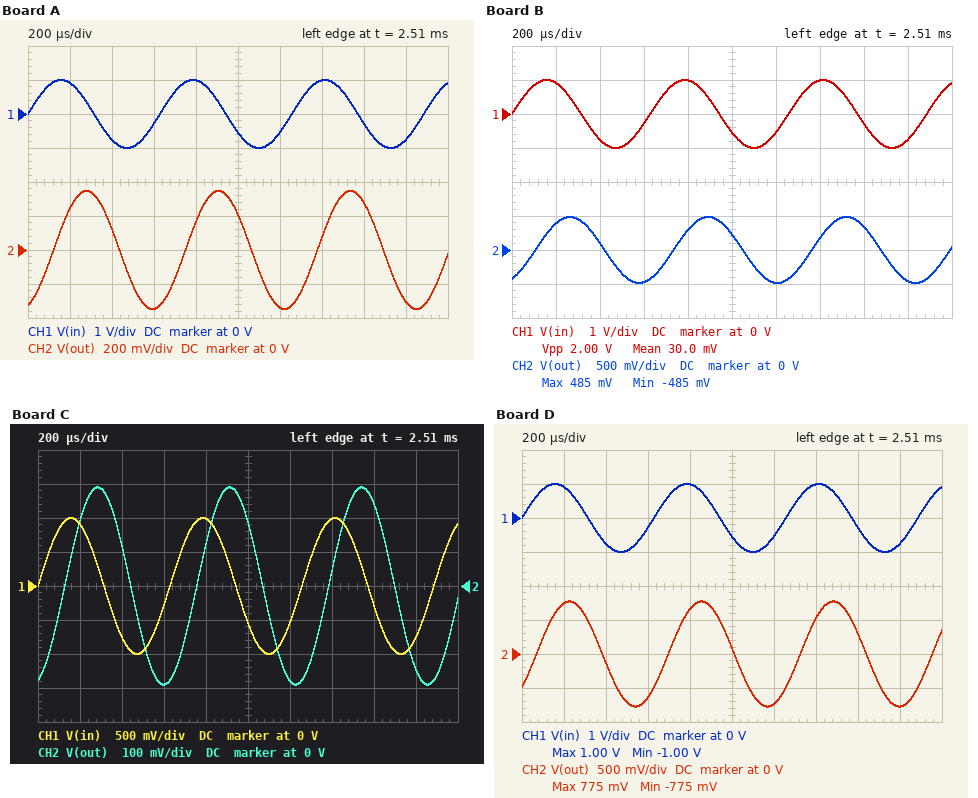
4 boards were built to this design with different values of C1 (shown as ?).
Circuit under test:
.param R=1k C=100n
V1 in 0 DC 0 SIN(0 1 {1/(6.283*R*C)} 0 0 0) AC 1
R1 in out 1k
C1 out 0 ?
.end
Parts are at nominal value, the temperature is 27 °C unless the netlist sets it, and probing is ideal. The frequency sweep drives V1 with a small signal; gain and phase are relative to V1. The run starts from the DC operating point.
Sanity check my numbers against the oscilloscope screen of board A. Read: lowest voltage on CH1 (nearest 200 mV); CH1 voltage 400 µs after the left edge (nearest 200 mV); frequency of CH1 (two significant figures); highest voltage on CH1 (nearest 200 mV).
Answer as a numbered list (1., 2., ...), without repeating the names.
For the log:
1. -1.0 V
2. -800 mV
3. 1.6 kHz
4. 1.0 V
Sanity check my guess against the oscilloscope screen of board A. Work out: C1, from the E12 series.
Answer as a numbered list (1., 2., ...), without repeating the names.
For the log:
1. 270 nF
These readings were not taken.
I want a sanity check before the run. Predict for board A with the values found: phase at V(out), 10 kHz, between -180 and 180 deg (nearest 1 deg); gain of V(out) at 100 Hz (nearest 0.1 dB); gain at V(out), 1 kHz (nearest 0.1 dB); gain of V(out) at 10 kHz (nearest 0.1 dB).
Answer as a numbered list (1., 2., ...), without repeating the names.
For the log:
1. -87 deg
2. -0.1 dB
3. -5.9 dB
4. -24.6 dB
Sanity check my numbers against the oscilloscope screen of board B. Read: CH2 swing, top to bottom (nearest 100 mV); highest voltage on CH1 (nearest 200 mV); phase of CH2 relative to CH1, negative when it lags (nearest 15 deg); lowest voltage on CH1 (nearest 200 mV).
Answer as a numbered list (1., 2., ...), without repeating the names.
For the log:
1. 1.0 V
2. 1.0 V
3. -60 deg
4. -1.0 V
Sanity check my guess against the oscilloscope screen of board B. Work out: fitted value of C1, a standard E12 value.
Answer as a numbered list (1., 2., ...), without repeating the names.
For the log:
1. 180 nF
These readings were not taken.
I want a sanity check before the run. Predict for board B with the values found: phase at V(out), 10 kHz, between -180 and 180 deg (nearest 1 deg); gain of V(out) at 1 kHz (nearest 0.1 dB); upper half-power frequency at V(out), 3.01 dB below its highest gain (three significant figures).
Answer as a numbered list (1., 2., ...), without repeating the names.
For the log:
1. -85 deg
2. -3.6 dB
3. 884 Hz
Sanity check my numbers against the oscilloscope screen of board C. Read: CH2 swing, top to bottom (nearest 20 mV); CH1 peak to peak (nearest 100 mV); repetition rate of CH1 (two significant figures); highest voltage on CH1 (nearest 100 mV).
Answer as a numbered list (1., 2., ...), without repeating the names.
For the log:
1. 580 mV
2. 2.0 V
3. 1.6 kHz
4. 1.0 V
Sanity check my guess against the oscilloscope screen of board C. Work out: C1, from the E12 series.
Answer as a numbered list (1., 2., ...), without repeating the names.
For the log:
1. 330 nF
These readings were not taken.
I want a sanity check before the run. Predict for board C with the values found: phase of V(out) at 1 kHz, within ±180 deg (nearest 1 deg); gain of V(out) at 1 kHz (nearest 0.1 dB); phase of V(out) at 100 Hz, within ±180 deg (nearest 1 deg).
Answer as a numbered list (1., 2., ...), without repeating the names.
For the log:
1. -64 deg
2. -7.2 dB
3. -12 deg
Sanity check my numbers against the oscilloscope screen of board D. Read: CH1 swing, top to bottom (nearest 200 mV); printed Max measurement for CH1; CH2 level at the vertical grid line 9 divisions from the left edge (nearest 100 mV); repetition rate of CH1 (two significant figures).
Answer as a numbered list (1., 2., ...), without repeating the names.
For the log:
1. 2.0 V
2. 1.00 V
3. -800 mV
4. 1.6 kHz
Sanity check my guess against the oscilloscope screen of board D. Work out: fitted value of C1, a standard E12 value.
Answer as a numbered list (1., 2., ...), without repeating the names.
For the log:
1. 82 nF
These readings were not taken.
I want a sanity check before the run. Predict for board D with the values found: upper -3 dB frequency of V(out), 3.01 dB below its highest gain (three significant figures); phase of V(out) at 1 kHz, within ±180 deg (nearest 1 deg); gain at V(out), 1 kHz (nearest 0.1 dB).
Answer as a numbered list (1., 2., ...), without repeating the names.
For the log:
1. 1.94 kHz
2. -27 deg
3. -1.0 dB
